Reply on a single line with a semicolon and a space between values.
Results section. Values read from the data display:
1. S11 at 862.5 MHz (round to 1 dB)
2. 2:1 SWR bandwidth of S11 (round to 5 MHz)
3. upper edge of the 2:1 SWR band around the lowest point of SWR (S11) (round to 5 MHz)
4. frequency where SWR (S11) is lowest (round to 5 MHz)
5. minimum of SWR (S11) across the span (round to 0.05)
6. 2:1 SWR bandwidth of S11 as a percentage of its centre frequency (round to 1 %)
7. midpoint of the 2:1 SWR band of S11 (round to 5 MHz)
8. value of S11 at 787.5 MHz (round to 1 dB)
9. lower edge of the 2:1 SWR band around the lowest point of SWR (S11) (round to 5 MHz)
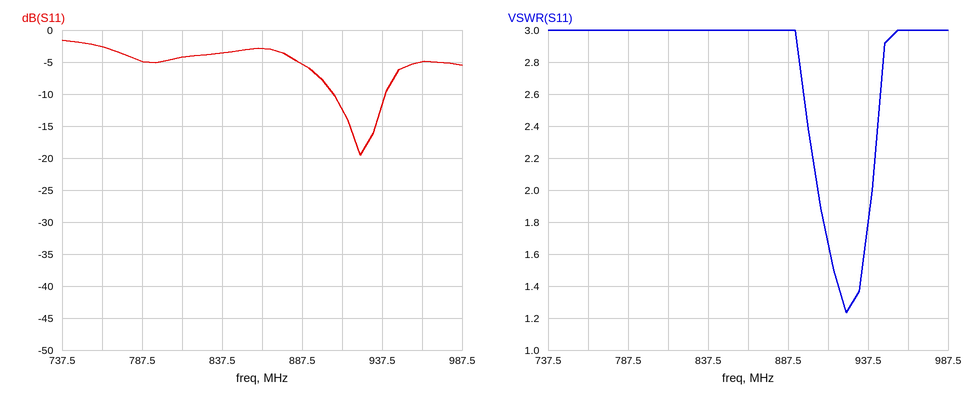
-3 dB; 35 MHz; 940 MHz; 925 MHz; 1.25; 4 %; 925 MHz; -5 dB; 905 MHz
